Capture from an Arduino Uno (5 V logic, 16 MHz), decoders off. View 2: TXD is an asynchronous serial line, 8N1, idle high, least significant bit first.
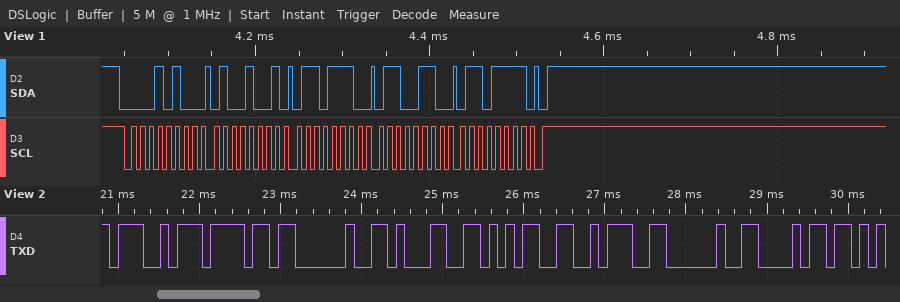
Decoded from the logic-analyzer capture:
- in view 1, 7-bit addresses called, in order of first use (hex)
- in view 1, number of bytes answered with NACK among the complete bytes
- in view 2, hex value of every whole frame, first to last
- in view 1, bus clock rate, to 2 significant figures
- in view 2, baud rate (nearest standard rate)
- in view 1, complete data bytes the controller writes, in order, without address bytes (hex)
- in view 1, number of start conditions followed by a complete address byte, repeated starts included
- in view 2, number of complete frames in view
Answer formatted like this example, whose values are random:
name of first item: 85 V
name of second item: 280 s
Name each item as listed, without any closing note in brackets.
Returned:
in view 1, 7-bit addresses called, in order of first use: 0x0A
in view 1, number of bytes answered with NACK among the complete bytes: 0
in view 2, hex value of every whole frame, first to last: A7 6F 20 31 35 3A 20 68
in view 1, bus clock rate, to 2 significant figures: 100 kHz
in view 2, baud rate: 9600 baud
in view 1, complete data bytes the controller writes, in order, without address bytes: 49 6E 66 6F
in view 1, number of start conditions followed by a complete address byte, repeated starts included: 1
in view 2, number of complete frames in view: 8
